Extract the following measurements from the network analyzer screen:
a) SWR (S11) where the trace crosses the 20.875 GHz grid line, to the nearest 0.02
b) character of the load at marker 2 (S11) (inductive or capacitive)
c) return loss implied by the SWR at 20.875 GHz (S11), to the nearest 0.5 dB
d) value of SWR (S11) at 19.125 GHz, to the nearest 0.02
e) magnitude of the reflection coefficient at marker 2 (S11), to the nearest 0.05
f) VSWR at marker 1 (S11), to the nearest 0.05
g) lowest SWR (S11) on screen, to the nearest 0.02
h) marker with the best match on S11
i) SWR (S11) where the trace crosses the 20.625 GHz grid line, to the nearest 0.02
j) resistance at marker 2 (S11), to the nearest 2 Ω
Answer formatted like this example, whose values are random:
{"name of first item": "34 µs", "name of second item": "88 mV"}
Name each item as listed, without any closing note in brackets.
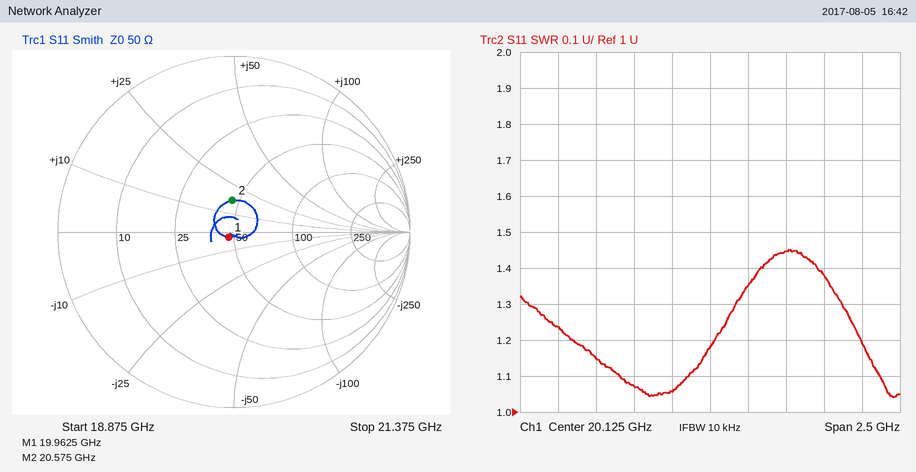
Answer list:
{"SWR (S11) where the trace crosses the 20.875 GHz grid line, to the nearest 0.02": "1.38", "character of the load at marker 2 (S11)": "inductive", "return loss implied by the SWR at 20.875 GHz (S11), to the nearest 0.5 dB": "16.0 dB", "value of SWR (S11) at 19.125 GHz, to the nearest 0.02": "1.24", "magnitude of the reflection coefficient at marker 2 (S11), to the nearest 0.05": "0.20", "VSWR at marker 1 (S11), to the nearest 0.05": "1.10", "lowest SWR (S11) on screen, to the nearest 0.02": "1.04", "marker with the best match on S11": "marker 1", "SWR (S11) where the trace crosses the 20.625 GHz grid line, to the nearest 0.02": "1.44", "resistance at marker 2 (S11), to the nearest 2 Ω": "46 Ω"}
